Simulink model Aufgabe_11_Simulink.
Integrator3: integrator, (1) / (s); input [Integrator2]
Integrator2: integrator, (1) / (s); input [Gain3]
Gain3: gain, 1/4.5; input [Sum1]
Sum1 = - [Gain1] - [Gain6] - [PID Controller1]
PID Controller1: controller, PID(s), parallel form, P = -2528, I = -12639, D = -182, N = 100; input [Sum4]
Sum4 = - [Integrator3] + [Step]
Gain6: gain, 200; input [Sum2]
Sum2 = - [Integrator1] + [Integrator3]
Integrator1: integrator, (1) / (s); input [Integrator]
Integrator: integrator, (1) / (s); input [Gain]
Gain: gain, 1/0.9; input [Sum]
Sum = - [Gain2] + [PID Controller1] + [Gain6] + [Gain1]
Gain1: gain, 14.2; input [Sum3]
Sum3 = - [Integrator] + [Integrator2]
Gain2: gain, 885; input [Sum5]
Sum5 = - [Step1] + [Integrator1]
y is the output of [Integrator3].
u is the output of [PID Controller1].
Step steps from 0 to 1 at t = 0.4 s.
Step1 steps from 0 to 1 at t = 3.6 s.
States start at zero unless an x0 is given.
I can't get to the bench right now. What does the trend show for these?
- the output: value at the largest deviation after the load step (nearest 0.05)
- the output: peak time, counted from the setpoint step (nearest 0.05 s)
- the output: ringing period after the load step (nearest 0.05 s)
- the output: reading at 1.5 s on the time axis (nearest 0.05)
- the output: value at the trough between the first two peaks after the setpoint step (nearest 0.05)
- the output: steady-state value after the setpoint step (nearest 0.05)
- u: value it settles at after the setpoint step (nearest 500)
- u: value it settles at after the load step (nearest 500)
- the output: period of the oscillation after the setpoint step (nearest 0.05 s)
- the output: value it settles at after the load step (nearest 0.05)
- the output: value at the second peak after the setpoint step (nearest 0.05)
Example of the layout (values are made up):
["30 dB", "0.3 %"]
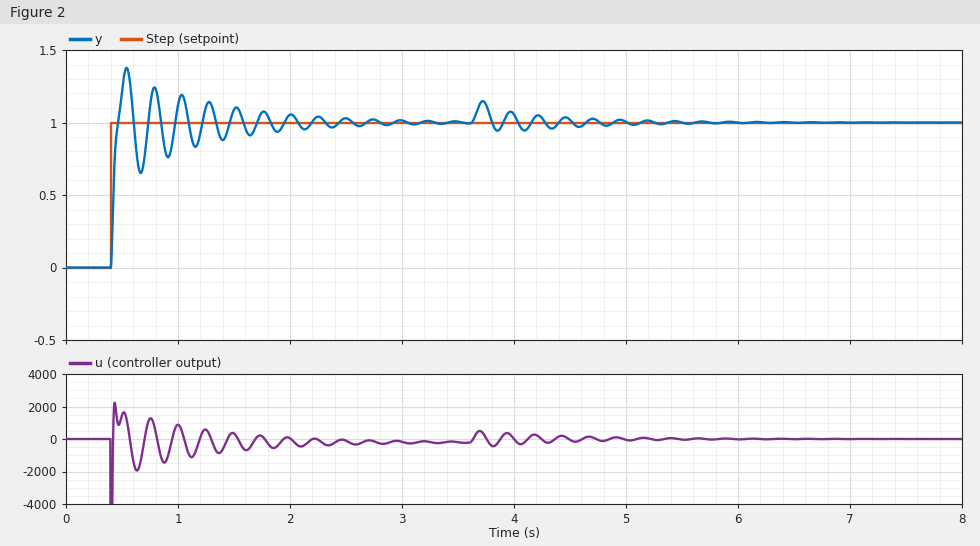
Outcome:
["1.15", "0.15 s", "0.25 s", "1.10", "0.65", "1.00", "0", "0", "0.25 s", "1.00", "1.25"]
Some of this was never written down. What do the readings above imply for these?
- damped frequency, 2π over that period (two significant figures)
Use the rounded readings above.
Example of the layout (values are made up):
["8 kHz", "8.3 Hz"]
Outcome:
["25 rad/s"]
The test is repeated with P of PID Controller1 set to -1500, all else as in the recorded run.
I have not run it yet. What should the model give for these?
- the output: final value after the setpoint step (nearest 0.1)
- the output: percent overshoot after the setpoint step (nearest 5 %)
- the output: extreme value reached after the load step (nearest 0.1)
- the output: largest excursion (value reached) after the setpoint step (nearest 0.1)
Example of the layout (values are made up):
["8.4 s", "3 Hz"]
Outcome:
["1.0", "35 %", "1.2", "1.4"]
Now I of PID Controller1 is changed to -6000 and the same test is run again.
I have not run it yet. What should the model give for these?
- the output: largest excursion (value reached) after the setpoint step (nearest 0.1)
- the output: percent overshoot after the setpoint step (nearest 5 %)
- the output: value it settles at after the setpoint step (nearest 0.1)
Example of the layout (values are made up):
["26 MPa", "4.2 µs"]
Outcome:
["1.3", "35 %", "1.0"]
